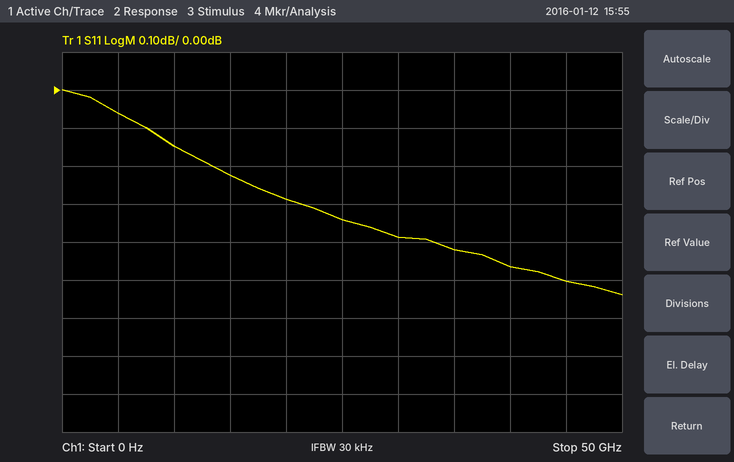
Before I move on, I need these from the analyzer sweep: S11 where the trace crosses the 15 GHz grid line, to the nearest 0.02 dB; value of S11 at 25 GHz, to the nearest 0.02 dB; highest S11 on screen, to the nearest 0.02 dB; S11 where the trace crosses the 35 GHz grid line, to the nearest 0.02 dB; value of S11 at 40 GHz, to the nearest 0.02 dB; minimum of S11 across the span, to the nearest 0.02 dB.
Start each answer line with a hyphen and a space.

- -0.22 dB
- -0.34 dB
- 0.00 dB
- -0.42 dB
- -0.46 dB
- -0.54 dB
